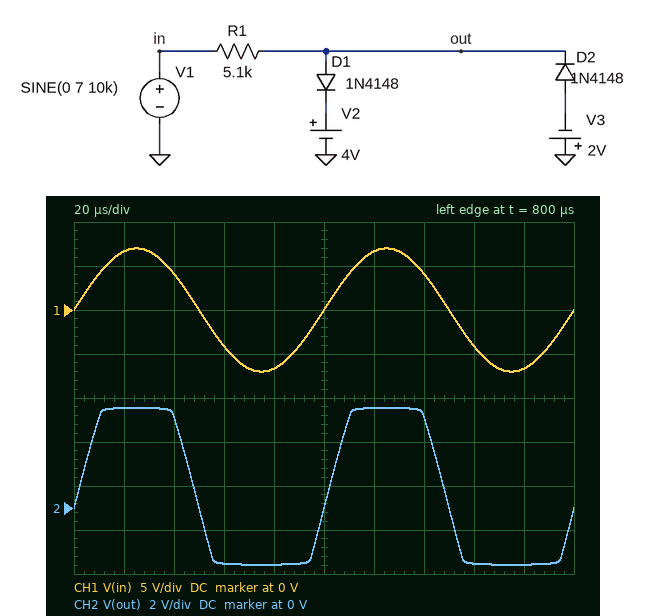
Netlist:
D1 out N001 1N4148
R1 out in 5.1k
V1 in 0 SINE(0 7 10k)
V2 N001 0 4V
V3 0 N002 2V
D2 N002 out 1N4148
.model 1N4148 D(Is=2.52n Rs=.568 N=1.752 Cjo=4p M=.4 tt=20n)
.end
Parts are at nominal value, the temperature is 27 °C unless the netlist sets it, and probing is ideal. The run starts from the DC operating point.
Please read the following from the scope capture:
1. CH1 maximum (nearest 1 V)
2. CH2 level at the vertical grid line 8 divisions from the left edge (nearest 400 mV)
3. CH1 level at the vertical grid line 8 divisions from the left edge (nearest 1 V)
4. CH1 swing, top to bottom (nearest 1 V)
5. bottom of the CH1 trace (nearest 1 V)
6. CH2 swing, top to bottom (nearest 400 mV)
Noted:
7 V
-2.4 V
-4 V
14 V
-7 V
7.2 V
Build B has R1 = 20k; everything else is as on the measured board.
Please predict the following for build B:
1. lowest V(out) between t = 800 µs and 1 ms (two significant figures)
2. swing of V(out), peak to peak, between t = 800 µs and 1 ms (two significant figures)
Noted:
-2.5 V
7.0 V
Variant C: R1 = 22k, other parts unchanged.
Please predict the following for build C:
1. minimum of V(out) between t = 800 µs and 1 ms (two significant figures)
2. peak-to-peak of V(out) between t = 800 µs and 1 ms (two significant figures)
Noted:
-2.5 V
7.0 V
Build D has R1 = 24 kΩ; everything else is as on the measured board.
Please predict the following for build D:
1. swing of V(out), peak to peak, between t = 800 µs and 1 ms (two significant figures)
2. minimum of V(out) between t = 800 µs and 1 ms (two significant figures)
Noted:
7.0 V
-2.5 V
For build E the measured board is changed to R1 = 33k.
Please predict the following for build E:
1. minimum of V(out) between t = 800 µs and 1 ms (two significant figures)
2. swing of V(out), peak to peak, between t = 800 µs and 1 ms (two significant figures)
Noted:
-2.5 V
7.0 V
